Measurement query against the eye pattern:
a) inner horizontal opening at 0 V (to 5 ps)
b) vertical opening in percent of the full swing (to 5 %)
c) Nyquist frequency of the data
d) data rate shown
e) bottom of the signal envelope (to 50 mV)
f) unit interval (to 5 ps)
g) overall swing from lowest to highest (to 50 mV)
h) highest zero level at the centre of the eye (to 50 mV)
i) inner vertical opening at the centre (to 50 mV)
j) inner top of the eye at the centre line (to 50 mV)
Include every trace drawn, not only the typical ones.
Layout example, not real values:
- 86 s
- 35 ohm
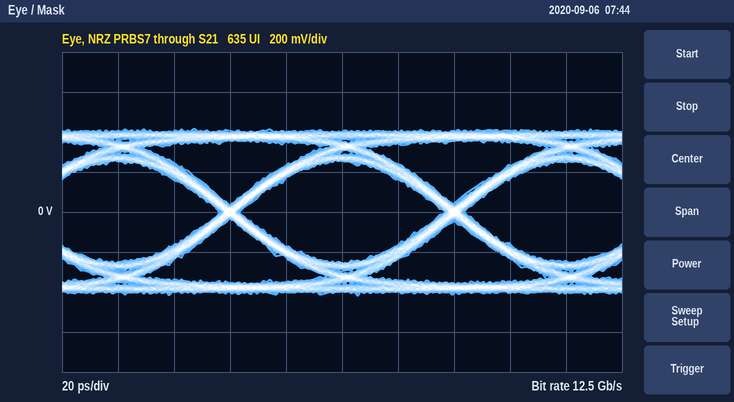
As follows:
- 75 ps
- 60 %
- 6.25 GHz
- 12.5 Gb/s
- -400 mV
- 80 ps
- 850 mV
- -250 mV
- 500 mV
- 250 mV
